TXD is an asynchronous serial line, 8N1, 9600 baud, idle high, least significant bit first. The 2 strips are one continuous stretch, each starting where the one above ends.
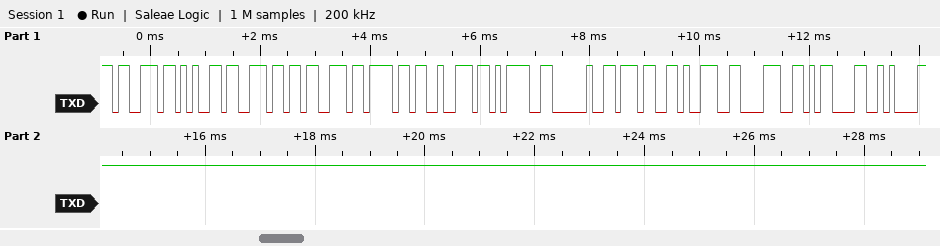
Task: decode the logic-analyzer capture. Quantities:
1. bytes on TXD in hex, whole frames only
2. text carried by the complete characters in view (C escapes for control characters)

0x73 0x65 0x6E 0x73 0x6F 0x72 0x3D 0x20 0x37 0x39 0x38 0x0D 0x0A
"sensor= 798\r\n"
